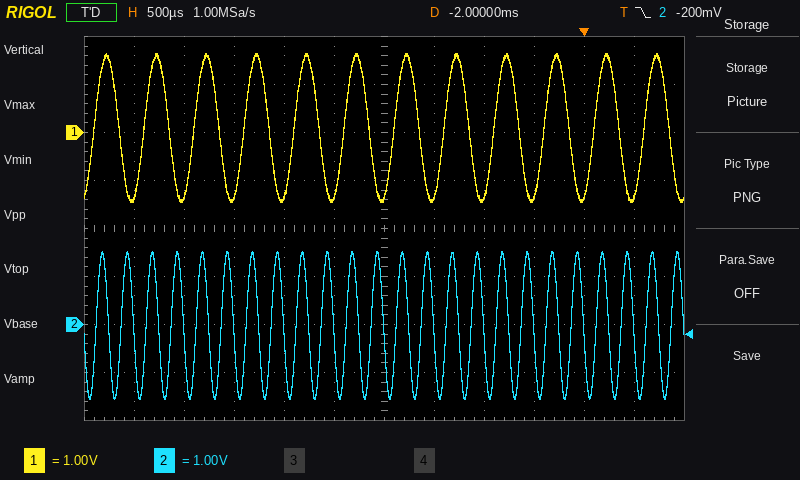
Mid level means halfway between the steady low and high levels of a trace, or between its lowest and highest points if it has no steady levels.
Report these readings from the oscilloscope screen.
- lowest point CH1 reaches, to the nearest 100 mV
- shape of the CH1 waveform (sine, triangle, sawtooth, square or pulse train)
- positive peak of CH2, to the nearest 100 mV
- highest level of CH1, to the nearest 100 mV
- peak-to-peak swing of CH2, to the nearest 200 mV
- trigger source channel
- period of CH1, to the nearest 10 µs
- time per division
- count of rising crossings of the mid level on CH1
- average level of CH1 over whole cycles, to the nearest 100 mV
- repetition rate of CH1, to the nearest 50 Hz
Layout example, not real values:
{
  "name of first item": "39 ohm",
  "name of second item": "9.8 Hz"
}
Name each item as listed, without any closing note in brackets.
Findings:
{
  "lowest point CH1 reaches, to the nearest 100 mV": "-1.4 V",
  "shape of the CH1 waveform": "sine",
  "positive peak of CH2, to the nearest 100 mV": "1.5 V",
  "highest level of CH1, to the nearest 100 mV": "1.6 V",
  "peak-to-peak swing of CH2, to the nearest 200 mV": "3.0 V",
  "trigger source channel": "CH2",
  "period of CH1, to the nearest 10 µs": "500 µs",
  "time per division": "500 µs",
  "count of rising crossings of the mid level on CH1": "12",
  "average level of CH1 over whole cycles, to the nearest 100 mV": "100 mV",
  "repetition rate of CH1, to the nearest 50 Hz": "2.00 kHz"
}
